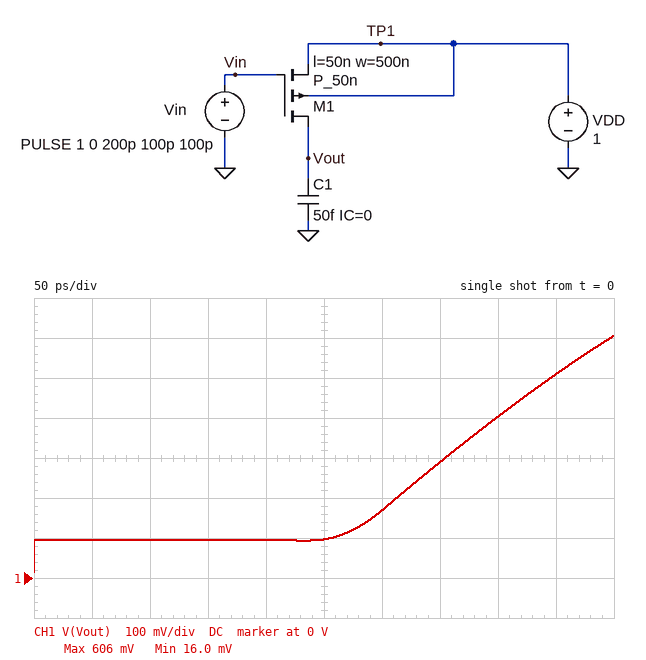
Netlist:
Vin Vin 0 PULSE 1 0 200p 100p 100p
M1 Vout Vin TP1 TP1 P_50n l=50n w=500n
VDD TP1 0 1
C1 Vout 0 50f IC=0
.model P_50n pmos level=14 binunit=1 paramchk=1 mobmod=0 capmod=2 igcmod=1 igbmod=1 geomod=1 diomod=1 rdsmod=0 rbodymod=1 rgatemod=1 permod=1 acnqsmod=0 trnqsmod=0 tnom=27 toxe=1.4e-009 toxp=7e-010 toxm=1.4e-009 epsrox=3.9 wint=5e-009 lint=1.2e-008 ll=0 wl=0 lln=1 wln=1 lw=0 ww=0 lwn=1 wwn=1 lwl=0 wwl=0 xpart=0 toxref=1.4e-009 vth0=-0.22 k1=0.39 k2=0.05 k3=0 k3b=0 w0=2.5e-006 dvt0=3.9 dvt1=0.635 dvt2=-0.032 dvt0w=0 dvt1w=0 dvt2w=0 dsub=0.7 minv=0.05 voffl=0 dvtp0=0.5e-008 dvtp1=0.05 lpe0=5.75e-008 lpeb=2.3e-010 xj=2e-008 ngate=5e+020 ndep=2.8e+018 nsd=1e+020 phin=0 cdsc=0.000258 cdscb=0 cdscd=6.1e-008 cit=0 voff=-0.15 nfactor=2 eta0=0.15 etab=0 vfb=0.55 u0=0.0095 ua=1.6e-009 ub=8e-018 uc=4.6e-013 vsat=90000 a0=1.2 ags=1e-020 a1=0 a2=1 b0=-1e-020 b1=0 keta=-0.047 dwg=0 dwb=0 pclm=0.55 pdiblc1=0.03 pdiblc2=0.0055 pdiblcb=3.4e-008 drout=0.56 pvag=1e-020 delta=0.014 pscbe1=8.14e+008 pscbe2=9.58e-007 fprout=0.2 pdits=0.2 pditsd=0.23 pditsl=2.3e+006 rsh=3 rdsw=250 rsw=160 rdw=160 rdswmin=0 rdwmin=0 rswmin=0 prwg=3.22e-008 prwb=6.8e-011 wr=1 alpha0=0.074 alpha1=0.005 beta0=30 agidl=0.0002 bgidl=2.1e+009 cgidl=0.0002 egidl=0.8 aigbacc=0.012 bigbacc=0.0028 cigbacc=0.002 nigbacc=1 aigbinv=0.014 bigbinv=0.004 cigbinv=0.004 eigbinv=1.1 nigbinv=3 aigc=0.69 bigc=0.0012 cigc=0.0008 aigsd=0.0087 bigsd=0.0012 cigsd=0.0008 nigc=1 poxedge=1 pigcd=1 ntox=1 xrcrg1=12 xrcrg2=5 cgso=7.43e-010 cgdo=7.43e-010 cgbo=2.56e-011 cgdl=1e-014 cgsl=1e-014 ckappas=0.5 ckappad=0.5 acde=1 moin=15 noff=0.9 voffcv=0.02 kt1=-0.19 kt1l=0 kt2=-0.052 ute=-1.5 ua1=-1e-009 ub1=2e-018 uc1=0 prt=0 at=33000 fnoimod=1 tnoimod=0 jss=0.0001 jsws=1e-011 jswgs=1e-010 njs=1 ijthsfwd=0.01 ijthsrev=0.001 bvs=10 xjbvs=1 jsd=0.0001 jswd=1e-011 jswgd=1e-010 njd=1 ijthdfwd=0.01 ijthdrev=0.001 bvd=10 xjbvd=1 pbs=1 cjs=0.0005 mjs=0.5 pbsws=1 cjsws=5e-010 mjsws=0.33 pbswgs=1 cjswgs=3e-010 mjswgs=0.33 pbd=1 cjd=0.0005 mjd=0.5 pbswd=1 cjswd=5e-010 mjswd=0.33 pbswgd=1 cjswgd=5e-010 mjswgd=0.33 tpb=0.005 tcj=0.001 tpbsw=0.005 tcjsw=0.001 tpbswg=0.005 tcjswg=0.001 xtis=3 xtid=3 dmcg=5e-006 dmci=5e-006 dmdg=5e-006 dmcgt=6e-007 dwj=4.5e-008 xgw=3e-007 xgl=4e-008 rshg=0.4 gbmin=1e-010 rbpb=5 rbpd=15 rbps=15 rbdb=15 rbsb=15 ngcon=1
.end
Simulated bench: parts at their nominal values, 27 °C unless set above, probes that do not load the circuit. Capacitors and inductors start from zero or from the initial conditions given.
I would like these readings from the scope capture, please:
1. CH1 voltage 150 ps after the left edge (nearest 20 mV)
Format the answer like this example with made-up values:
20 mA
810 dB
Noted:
100 mV
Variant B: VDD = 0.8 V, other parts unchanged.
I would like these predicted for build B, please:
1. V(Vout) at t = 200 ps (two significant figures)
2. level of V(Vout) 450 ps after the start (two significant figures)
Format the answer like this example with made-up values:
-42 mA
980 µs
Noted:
79 mV
340 mV
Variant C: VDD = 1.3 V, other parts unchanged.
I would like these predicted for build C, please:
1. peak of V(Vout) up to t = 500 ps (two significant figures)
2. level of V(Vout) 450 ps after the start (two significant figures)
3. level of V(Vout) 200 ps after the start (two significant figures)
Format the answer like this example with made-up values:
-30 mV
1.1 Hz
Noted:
910 mV
790 mV
130 mV
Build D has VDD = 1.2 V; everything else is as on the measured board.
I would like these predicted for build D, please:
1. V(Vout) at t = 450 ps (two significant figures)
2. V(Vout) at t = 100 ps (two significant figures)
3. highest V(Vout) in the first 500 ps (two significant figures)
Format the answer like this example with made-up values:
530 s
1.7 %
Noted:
690 mV
110 mV
800 mV
